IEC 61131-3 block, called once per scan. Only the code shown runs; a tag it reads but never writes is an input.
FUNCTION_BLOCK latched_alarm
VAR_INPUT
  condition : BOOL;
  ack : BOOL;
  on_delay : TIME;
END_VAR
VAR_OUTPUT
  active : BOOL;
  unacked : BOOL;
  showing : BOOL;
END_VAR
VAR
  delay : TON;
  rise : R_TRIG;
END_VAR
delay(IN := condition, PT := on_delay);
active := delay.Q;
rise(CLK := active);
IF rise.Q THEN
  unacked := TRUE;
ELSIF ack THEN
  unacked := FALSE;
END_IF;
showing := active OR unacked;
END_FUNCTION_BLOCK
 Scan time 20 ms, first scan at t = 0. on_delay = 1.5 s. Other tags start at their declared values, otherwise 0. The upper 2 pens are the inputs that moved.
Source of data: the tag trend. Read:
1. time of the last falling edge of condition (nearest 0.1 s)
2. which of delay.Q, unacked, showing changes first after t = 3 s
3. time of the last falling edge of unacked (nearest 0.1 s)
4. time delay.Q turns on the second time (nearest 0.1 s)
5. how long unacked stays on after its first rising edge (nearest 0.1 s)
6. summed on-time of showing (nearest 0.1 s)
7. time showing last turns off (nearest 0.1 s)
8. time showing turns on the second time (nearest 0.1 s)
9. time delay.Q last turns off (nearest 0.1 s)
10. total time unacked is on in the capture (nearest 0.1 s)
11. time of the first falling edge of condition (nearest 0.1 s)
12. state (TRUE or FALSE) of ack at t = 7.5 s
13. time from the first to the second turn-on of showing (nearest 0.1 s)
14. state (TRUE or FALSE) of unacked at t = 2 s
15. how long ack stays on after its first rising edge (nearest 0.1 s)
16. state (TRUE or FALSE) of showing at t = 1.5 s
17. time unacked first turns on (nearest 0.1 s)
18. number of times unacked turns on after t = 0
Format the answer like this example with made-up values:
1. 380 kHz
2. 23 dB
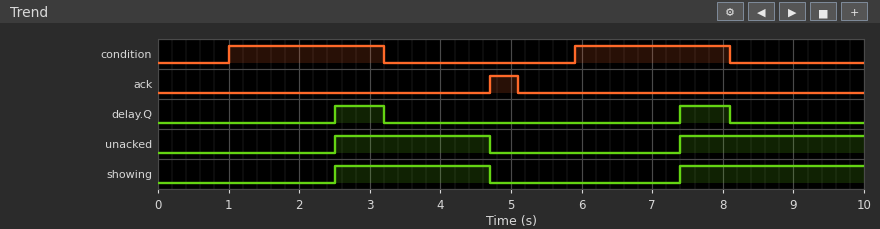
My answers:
1. 8.1 s
2. delay.Q
3. 4.7 s
4. 7.4 s
5. 2.2 s
6. 4.8 s
7. 4.7 s
8. 7.4 s
9. 8.1 s
10. 4.8 s
11. 3.2 s
12. FALSE
13. 4.9 s
14. FALSE
15. 0.4 s
16. FALSE
17. 2.5 s
18. 2
